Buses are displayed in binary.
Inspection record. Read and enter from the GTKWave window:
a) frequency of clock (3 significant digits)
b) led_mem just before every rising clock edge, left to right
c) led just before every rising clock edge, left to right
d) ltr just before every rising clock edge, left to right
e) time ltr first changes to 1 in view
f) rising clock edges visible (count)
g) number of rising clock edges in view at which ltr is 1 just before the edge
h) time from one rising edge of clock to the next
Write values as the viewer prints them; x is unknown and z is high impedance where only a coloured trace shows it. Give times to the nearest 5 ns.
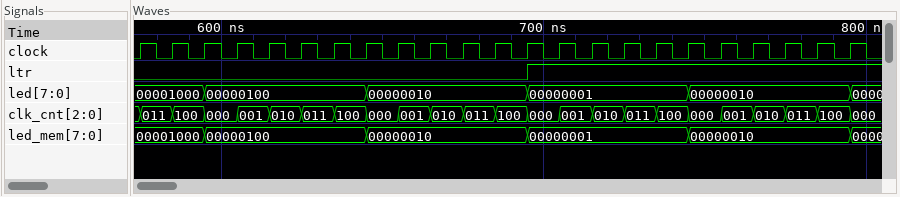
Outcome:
100 MHz
00001000, 00001000, 00001000, 00000100, 00000100, 00000100, 00000100, 00000100, 00000010, 00000010, 00000010, 00000010, 00000010, 00000001, 00000001, 00000001, 00000001, 00000001, 00000010, 00000010, 00000010, 00000010, 00000010
00001000, 00001000, 00001000, 00000100, 00000100, 00000100, 00000100, 00000100, 00000010, 00000010, 00000010, 00000010, 00000010, 00000001, 00000001, 00000001, 00000001, 00000001, 00000010, 00000010, 00000010, 00000010, 00000010
0 0 0 0 0 0 0 0 0 0 0 0 0 1 1 1 1 1 1 1 1 1 1
695 ns
23
10
10 ns
